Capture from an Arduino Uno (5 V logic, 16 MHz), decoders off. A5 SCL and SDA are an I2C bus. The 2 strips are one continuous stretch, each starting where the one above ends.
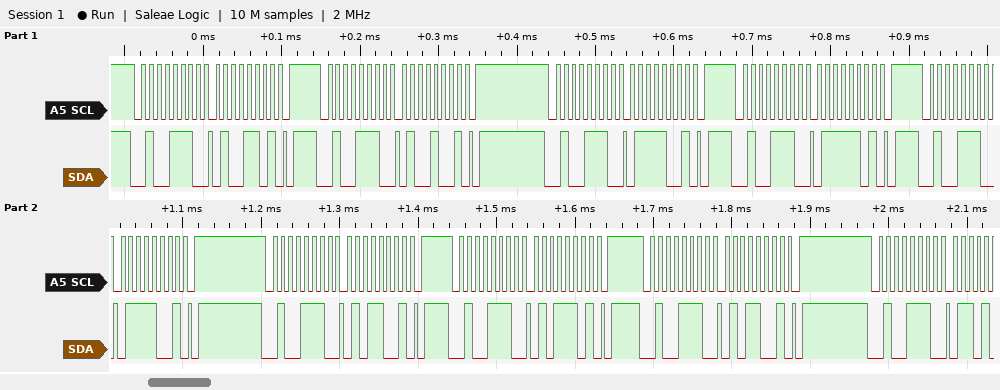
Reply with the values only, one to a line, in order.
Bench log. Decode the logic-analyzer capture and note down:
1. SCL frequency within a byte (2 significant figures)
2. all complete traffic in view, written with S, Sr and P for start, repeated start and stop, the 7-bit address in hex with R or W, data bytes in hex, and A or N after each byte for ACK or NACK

100 kHz
S 27W A 4D A P S 27W A 49 A P S 27W A 79 A P S 27W A 7D A P S 27W A 79 A P S 27W A 59 A P S 27W A 5D A P S 27W A 59 A P S 27W A
